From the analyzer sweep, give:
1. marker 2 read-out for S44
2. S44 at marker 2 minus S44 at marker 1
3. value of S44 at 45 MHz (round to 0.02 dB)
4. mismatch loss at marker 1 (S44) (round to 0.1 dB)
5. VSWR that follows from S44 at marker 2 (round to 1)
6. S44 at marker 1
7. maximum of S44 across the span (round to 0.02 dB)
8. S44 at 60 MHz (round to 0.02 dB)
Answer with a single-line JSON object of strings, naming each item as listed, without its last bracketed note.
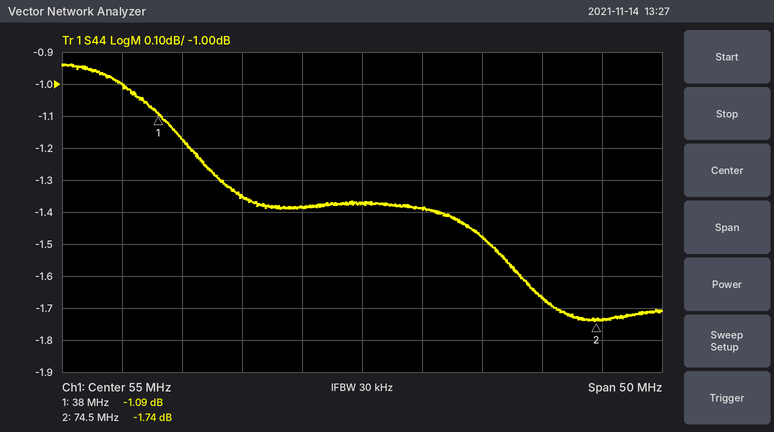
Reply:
{"marker 2 read-out for S44": "-1.74 dB", "S44 at marker 2 minus S44 at marker 1": "-0.65 dB", "value of S44 at 45 MHz": "-1.36 dB", "mismatch loss at marker 1 (S44)": "6.5 dB", "VSWR that follows from S44 at marker 2": "10", "S44 at marker 1": "-1.09 dB", "maximum of S44 across the span": "-0.94 dB", "S44 at 60 MHz": "-1.38 dB"}
